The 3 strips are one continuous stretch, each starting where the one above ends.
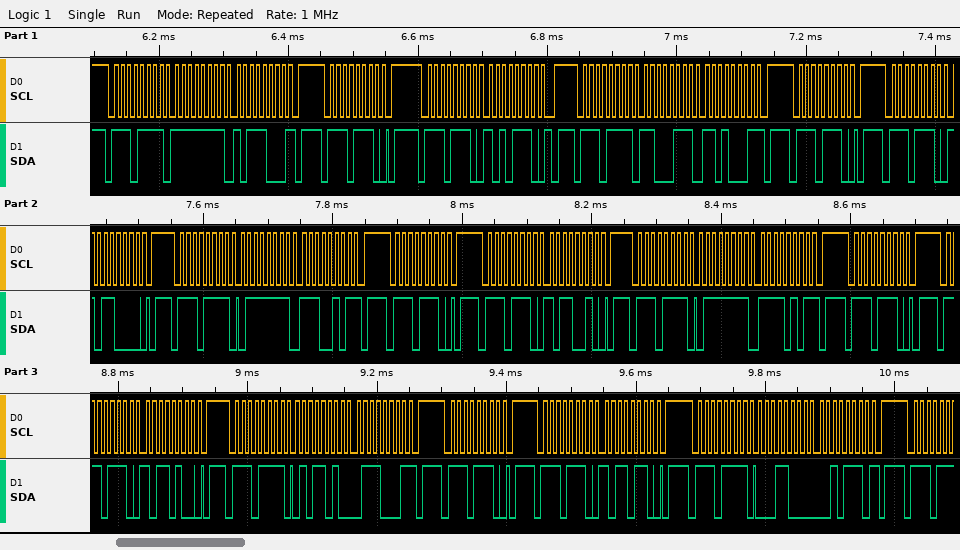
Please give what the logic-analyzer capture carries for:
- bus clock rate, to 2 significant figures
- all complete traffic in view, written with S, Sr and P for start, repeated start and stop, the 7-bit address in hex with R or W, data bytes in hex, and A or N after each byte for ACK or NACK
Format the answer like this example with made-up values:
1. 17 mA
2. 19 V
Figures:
1. 100 kHz
2. S 77R A FF A B8 N P S 77W A P S 77W A AE A P S 77R A C7 A D1 N P S 77W A P S 77W A B0 A P S 77R A 7F A E5 N P S 77W A P S 77W A B2 A P S 77R A 7F A F5 N P S 77W A P S 77W A B4 A P S 77R A 5A A 71 N P S 77W A P S 77W A B6 A P S 77R A 18 A 2E N P
